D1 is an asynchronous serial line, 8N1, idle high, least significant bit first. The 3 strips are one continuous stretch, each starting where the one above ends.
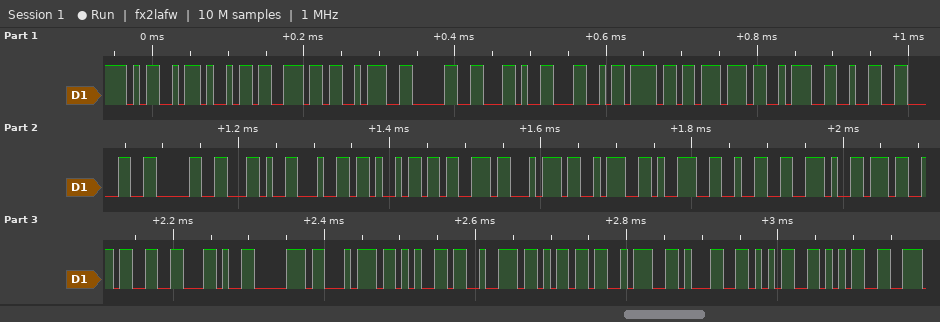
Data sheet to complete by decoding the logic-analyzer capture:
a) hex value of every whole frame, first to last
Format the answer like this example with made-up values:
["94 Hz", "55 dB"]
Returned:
["4D 69 6E 3A 30 2C 4C 6F 77 3A 32 30 30 2C 64 69 73 74 3A 39 32 2E 37 33 2C 70 74 65 72 6D 3A 31 35 35"]
